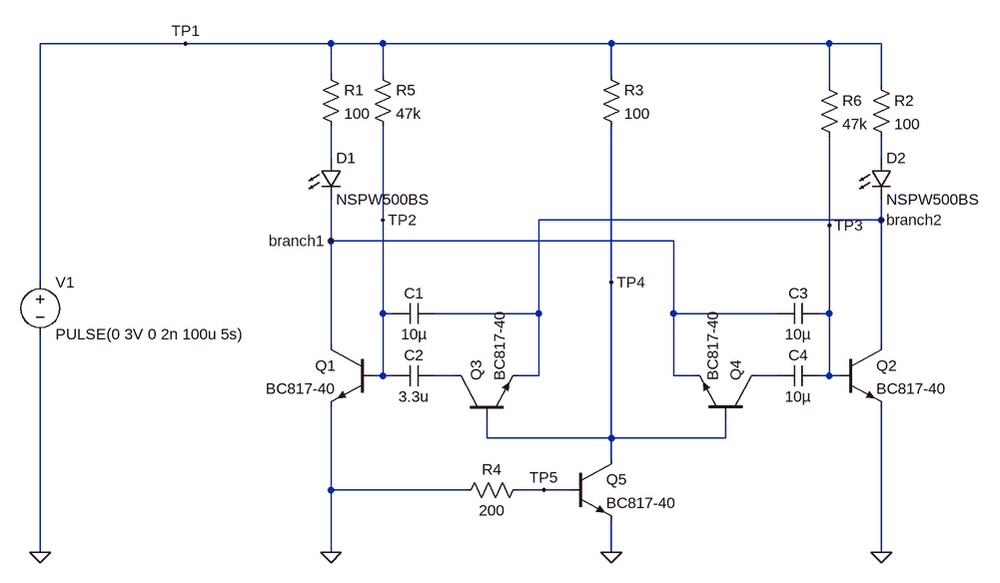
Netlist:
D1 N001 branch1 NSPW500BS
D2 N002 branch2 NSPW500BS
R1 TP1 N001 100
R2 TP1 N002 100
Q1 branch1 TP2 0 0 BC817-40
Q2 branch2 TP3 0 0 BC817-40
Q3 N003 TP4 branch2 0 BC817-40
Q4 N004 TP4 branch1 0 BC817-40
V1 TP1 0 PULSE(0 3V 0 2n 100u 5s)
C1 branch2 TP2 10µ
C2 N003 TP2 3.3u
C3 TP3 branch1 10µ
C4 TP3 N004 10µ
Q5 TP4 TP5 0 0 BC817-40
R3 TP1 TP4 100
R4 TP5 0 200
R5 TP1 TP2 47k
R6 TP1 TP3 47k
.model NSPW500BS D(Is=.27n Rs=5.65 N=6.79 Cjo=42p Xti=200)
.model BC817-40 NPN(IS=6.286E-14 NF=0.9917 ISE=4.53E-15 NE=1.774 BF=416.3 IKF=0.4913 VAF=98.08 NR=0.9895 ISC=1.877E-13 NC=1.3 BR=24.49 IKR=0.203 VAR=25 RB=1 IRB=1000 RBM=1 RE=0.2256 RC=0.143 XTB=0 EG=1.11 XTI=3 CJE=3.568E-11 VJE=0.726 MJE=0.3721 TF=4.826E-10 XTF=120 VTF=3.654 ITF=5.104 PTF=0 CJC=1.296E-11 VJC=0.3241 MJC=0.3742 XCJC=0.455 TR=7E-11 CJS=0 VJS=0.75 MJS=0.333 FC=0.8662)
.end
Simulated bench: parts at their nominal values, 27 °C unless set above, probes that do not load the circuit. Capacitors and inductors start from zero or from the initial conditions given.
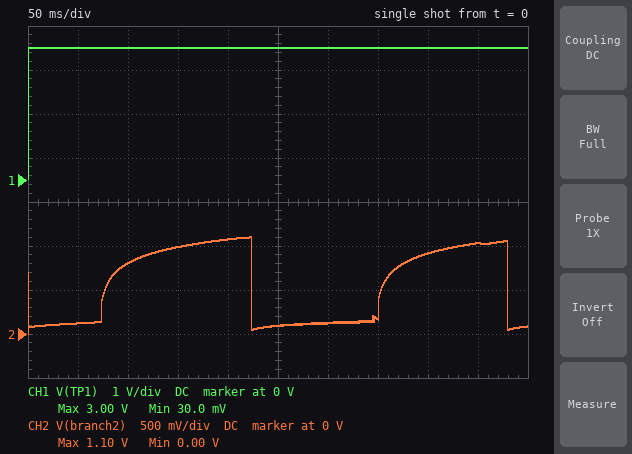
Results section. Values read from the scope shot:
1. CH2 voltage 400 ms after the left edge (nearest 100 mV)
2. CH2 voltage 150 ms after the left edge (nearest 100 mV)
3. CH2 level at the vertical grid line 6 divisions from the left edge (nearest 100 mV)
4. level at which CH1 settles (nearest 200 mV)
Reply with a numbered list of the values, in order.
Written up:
1. 900 mV
2. 1.0 V
3. 100 mV
4. 3.0 V
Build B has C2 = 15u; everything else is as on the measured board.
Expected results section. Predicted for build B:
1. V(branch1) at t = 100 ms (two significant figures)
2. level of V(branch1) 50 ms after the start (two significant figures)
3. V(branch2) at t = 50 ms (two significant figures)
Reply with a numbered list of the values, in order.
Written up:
1. 150 mV
2. 120 mV
3. 970 mV
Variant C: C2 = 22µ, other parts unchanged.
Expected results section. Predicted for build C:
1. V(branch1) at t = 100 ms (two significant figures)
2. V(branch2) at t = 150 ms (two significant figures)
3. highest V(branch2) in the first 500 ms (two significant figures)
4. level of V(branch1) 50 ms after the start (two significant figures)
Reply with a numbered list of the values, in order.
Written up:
1. 150 mV
2. 110 mV
3. 1.1 V
4. 120 mV
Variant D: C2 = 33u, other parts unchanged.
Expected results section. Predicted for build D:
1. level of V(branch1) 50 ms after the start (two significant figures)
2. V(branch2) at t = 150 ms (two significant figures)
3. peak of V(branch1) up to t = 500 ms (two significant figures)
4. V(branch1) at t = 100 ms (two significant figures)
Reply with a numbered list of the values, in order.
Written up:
1. 120 mV
2. 110 mV
3. 1.2 V
4. 150 mV
